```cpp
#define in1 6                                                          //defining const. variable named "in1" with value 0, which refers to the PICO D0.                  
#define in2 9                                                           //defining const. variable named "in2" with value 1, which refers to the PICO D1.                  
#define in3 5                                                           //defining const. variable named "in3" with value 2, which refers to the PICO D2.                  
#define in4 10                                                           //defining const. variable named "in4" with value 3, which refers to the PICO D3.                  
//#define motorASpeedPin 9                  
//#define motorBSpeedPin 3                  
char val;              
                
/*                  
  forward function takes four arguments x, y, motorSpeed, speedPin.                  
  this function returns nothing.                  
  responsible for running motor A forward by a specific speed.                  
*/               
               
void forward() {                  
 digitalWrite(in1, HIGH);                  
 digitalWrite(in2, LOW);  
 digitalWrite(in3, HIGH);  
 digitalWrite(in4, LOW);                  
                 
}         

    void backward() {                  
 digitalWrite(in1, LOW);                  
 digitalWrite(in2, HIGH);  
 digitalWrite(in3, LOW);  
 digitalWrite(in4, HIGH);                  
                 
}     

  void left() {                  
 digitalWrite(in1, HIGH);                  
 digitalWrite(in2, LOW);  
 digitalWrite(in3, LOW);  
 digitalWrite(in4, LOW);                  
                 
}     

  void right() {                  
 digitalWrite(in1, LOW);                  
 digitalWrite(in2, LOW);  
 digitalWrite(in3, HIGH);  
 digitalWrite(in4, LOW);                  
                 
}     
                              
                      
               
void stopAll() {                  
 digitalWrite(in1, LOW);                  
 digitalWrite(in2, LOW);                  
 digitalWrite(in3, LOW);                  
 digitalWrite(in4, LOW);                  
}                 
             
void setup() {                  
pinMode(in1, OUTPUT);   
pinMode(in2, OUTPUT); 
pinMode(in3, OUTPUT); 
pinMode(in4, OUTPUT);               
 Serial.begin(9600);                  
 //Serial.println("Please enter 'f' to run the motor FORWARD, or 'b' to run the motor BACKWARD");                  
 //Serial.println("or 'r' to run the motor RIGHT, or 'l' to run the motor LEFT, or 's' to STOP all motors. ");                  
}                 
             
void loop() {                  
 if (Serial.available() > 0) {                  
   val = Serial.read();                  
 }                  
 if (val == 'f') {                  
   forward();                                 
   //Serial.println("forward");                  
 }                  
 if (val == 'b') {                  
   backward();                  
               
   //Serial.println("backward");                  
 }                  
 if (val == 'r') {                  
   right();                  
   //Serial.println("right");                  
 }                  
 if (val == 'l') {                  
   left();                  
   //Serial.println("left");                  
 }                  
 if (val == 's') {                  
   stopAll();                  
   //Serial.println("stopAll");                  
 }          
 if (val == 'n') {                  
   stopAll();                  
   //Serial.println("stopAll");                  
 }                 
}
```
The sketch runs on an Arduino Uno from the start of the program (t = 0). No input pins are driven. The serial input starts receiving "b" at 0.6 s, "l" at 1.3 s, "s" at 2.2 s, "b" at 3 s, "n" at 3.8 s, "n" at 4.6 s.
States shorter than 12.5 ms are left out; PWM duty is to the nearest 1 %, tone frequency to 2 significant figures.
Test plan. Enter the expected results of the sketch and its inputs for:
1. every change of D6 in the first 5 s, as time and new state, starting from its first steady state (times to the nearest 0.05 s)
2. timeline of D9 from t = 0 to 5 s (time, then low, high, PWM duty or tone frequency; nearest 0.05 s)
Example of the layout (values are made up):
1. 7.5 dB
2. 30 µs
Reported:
1. 0 s low; 1.3 s high; 2.2 s low
2. 0 s low; 0.6 s high; 1.3 s low; 3 s high; 3.8 s low
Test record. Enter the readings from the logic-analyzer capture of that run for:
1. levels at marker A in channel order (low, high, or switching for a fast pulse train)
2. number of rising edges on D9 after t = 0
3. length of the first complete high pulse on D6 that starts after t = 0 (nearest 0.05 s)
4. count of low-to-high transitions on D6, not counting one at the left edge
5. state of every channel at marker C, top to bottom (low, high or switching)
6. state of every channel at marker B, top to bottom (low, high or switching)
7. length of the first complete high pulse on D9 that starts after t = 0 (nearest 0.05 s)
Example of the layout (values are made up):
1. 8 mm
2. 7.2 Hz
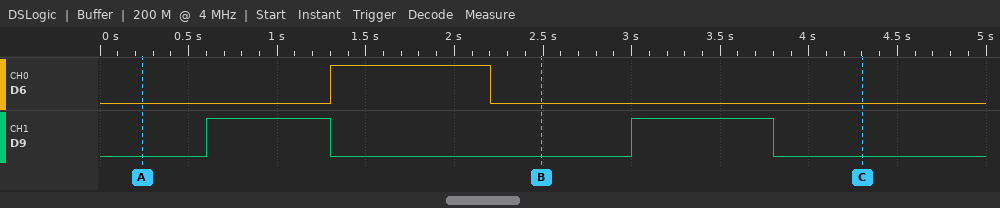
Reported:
1. D6 low, D9 low
2. 2
3. 0.90 s
4. 1
5. D6 low, D9 low
6. D6 low, D9 low
7. 0.70 s
